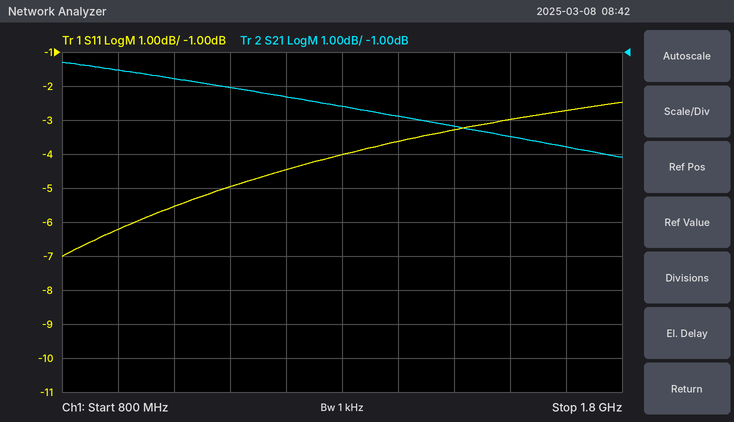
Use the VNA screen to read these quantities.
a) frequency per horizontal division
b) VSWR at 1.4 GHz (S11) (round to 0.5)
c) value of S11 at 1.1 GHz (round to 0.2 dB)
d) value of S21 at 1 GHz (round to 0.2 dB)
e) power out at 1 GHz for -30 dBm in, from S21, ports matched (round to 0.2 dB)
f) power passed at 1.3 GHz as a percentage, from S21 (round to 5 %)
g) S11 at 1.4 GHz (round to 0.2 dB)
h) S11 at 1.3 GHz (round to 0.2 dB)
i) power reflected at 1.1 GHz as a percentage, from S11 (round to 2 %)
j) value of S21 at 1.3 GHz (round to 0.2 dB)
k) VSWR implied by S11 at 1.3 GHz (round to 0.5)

100 MHz
5.0
-5.0 dB
-1.8 dB
-31.8 dBm
55 %
-3.6 dB
-4.0 dB
32 %
-2.6 dB
4.5
